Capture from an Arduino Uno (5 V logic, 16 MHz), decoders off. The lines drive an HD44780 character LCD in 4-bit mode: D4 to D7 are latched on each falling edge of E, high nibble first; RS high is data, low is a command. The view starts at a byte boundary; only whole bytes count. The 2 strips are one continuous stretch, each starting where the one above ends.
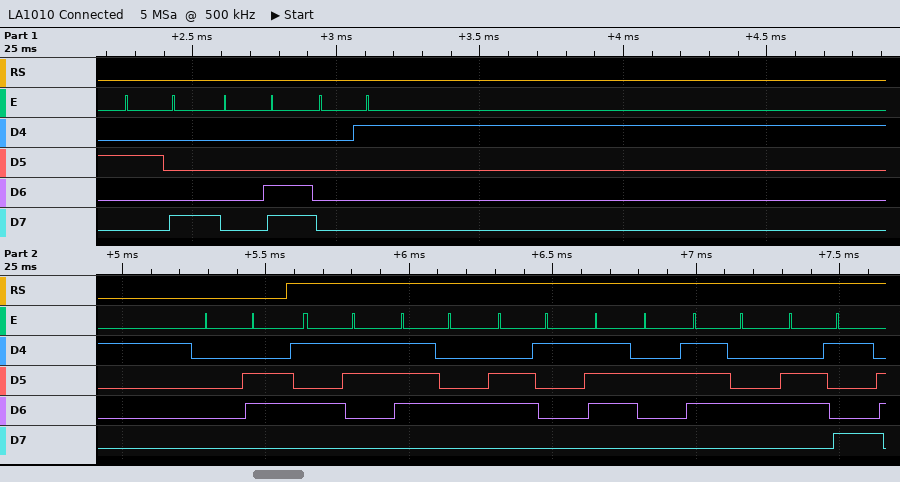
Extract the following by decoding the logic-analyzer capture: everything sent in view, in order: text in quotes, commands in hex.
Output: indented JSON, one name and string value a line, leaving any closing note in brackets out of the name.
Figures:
{
  "everything sent in view, in order: text in quotes, commands in hex": "0x28 0x0C 0x01 0x06 \"Starti\""
}
